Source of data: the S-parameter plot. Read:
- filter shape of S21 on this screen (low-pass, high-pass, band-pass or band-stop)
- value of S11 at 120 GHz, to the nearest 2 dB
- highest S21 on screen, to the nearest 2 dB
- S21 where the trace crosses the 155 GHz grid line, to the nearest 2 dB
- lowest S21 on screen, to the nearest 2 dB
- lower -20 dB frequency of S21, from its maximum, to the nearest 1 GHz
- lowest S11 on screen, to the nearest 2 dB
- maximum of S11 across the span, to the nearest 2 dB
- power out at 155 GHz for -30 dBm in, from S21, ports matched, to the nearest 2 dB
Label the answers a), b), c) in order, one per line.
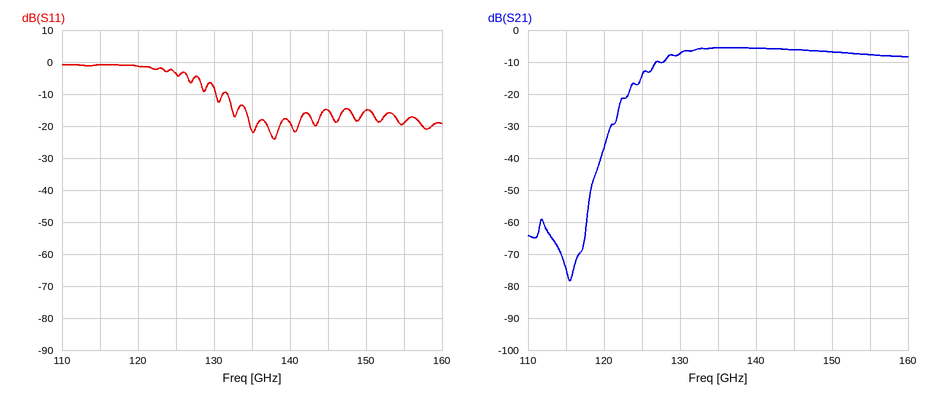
a) high-pass
b) -2 dB
c) -6 dB
d) -8 dB
e) -78 dB
f) 122 GHz
g) -24 dB
h) 0 dB
i) -38 dBm
